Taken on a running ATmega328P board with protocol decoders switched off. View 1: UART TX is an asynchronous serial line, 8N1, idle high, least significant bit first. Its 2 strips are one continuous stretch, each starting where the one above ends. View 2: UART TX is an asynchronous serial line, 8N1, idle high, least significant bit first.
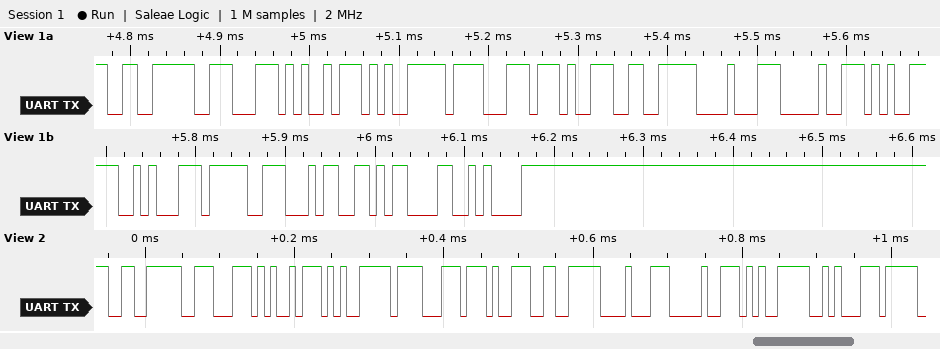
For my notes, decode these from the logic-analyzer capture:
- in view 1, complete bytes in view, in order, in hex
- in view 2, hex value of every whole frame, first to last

E6 8E A5 E5 8F 97 E6 88 90 E5 8A 9F 34 0D 0A
E6 8E A5 E5 8F 97 E6 88 90 E5 8A
